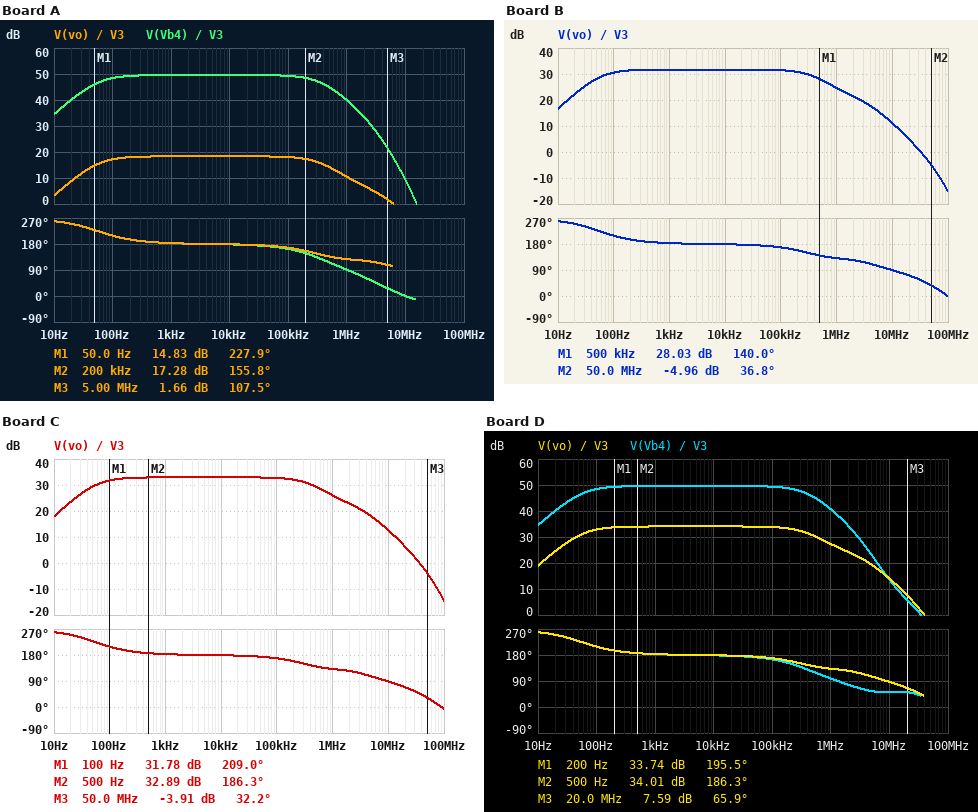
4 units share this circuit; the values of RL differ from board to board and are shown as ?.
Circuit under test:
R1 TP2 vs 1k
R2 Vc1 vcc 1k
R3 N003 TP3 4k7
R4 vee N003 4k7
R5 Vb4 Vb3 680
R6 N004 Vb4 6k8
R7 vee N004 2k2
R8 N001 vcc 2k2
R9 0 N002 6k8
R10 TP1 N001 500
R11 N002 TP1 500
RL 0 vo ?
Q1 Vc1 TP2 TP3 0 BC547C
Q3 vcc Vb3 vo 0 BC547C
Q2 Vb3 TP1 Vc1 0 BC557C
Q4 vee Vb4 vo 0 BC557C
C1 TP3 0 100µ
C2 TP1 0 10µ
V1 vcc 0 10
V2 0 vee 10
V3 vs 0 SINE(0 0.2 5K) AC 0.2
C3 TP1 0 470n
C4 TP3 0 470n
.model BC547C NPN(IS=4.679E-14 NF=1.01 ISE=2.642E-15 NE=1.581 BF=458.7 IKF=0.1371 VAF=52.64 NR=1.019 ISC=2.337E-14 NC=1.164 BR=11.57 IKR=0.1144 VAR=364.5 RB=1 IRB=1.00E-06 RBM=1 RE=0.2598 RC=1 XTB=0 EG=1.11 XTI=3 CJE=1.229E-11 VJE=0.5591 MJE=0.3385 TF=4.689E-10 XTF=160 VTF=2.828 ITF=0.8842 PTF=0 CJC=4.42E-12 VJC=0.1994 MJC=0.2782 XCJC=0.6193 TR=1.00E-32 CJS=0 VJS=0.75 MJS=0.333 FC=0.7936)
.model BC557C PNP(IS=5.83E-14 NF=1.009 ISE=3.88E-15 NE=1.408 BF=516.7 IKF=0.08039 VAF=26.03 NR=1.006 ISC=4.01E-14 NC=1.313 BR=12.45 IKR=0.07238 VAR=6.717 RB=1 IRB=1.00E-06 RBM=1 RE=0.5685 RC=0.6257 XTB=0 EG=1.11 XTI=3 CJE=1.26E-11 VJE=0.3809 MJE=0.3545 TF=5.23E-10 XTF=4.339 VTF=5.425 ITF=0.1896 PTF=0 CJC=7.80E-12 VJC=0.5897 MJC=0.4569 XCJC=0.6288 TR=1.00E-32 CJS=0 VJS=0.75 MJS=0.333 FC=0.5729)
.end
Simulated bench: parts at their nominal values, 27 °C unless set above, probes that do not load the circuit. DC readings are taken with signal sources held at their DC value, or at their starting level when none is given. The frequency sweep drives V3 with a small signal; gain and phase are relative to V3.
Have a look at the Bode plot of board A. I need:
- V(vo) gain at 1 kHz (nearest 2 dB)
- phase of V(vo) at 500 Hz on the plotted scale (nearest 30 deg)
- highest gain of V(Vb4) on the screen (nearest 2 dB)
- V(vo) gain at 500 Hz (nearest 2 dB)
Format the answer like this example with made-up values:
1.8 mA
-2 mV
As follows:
18 dB
180 deg
50 dB
18 dB
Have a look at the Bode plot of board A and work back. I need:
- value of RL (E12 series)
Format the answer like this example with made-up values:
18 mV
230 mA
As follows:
68 Ω
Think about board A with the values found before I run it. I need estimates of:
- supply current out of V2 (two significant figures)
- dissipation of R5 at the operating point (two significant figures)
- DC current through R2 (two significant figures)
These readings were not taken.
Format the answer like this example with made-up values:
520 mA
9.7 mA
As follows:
2.1 mA
800 µW
2.1 mA
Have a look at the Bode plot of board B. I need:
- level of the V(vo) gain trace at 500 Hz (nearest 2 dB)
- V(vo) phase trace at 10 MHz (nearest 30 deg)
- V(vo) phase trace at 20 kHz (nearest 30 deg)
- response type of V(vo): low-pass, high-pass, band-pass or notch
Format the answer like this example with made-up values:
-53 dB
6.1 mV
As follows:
32 dB
90 deg
180 deg
band-pass
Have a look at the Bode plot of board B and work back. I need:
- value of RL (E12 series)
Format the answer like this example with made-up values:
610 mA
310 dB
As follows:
390 Ω
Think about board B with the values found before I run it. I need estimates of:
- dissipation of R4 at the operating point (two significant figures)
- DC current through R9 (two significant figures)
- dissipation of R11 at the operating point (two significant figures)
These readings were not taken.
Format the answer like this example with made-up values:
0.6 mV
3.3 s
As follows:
4.7 mW
1.0 mA
500 µW
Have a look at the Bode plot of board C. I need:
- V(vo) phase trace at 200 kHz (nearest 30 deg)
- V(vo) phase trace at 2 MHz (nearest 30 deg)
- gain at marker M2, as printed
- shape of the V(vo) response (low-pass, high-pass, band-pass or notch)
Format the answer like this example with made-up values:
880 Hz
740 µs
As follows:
150 deg
120 deg
32.89 dB
band-pass
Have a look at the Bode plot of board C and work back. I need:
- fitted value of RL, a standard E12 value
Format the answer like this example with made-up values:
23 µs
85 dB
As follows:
470 Ω
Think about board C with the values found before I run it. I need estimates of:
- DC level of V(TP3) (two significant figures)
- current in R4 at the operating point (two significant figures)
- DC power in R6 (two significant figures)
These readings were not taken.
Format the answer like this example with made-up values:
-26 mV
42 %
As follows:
-620 mV
1.0 mA
8.0 mW
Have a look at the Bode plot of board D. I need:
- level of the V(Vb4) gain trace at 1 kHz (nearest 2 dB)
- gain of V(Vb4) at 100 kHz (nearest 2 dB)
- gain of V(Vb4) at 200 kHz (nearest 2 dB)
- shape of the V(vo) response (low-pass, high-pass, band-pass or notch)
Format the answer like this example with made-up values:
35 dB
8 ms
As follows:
50 dB
50 dB
48 dB
band-pass
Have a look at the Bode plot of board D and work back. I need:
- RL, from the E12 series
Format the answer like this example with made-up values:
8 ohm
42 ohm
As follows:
560 Ω
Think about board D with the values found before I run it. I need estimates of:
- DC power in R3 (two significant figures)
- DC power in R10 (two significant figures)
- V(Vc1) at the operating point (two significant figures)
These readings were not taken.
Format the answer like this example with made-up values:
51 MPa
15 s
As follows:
4.7 mW
500 µW
7.9 V
